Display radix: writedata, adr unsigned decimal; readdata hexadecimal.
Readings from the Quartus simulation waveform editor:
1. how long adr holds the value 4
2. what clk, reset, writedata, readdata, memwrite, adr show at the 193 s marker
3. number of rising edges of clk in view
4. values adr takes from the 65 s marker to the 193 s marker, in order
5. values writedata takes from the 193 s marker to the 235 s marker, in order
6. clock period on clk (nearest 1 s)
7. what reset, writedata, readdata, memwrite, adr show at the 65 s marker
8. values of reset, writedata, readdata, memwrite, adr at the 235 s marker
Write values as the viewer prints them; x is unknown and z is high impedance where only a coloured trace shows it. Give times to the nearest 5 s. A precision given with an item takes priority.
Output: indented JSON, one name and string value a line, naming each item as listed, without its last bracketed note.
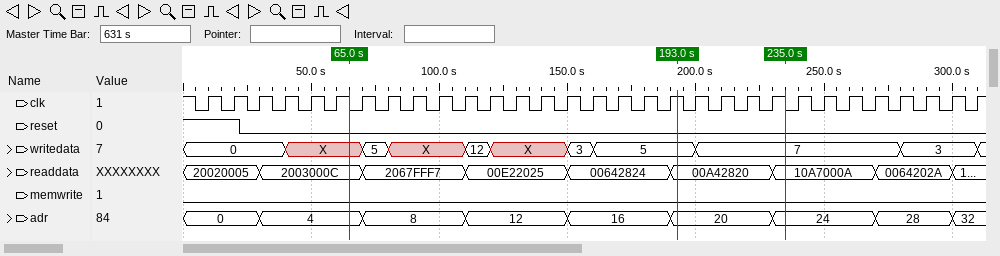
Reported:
{
  "how long adr holds the value 4": "40 s",
  "what clk, reset, writedata, readdata, memwrite, adr show at the 193 s marker": "clk=1, reset=0, writedata=5, readdata=00A42820, memwrite=0, adr=20",
  "number of rising edges of clk in view": "31",
  "values adr takes from the 65 s marker to the 193 s marker, in order": "4, 8, 12, 16, 20",
  "values writedata takes from the 193 s marker to the 235 s marker, in order": "5, 7",
  "clock period on clk": "10 s",
  "what reset, writedata, readdata, memwrite, adr show at the 65 s marker": "reset=0, writedata=X, readdata=2003000C, memwrite=0, adr=4",
  "values of reset, writedata, readdata, memwrite, adr at the 235 s marker": "reset=0, writedata=7, readdata=10A7000A, memwrite=0, adr=24"
}
